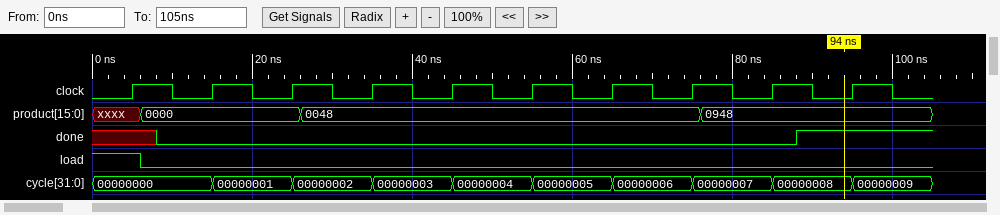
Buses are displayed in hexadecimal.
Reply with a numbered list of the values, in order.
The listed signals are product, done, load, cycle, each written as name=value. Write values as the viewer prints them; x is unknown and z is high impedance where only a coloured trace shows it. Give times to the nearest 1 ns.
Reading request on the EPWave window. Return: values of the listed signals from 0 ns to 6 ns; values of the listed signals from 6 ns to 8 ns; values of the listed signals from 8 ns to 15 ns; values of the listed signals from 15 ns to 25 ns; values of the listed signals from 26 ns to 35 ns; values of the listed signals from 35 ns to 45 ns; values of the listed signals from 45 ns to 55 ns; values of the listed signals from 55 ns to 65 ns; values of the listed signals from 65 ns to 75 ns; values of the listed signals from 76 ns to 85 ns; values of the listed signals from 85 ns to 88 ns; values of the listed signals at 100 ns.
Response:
1. product=xxxx, done=x, load=1, cycle=00000000
2. product=0000, done=x, load=0, cycle=00000000
3. product=0000, done=0, load=0, cycle=00000000
4. product=0000, done=0, load=0, cycle=00000001
5. product=0048, done=0, load=0, cycle=00000002
6. product=0048, done=0, load=0, cycle=00000003
7. product=0048, done=0, load=0, cycle=00000004
8. product=0048, done=0, load=0, cycle=00000005
9. product=0048, done=0, load=0, cycle=00000006
10. product=0948, done=0, load=0, cycle=00000007
11. product=0948, done=0, load=0, cycle=00000008
12. product=0948, done=1, load=0, cycle=00000009
